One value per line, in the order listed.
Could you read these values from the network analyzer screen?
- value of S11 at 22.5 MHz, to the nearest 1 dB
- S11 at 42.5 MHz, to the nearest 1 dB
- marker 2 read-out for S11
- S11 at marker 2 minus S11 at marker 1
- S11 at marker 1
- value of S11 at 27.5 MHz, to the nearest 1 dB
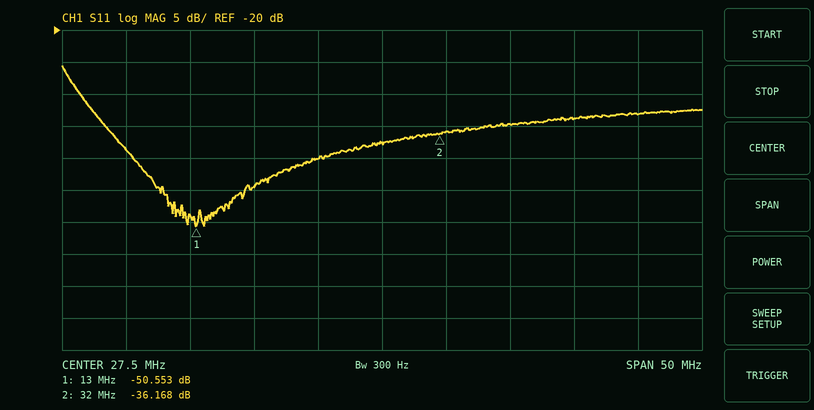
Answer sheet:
-40 dB
-34 dB
-36.168 dB
14.385 dB
-50.553 dB
-38 dB
